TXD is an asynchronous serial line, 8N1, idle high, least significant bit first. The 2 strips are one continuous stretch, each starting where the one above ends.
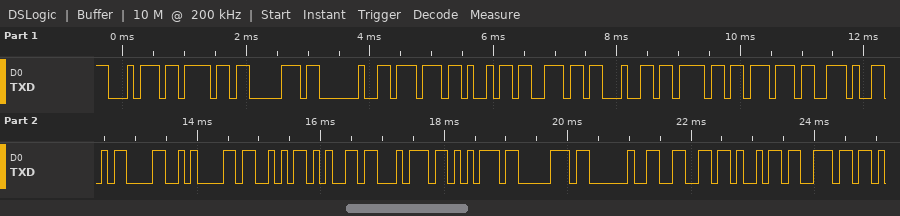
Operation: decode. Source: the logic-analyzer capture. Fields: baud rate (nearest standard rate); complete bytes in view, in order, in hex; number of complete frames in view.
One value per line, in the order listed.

9600 baud
74 6F 70 20 77 69 6E 64 6F 77 2E 0D 0A 53 65 74 75 70 20 66 69 6E
22
